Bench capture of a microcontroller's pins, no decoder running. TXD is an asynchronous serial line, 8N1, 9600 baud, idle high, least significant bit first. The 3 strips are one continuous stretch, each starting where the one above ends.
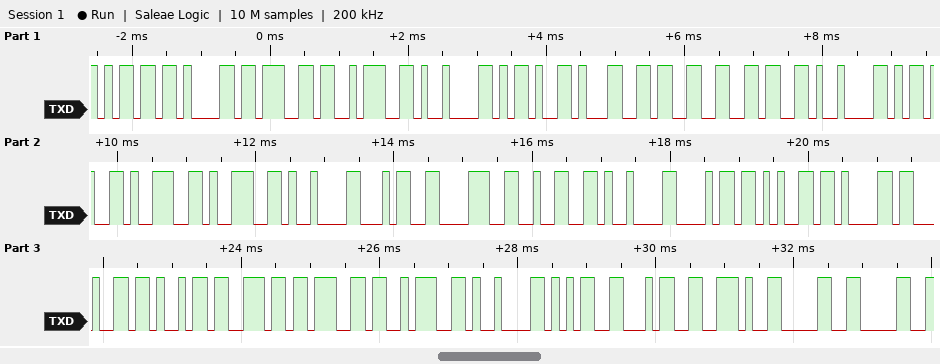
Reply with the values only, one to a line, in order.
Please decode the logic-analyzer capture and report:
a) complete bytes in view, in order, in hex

6D 61 67 3A 09 2D 31 33 36 09 2D 39 39 09 34 38 32 09 68 65 61 64 69 6E 67 3A 09 35 34 2E 30 30
